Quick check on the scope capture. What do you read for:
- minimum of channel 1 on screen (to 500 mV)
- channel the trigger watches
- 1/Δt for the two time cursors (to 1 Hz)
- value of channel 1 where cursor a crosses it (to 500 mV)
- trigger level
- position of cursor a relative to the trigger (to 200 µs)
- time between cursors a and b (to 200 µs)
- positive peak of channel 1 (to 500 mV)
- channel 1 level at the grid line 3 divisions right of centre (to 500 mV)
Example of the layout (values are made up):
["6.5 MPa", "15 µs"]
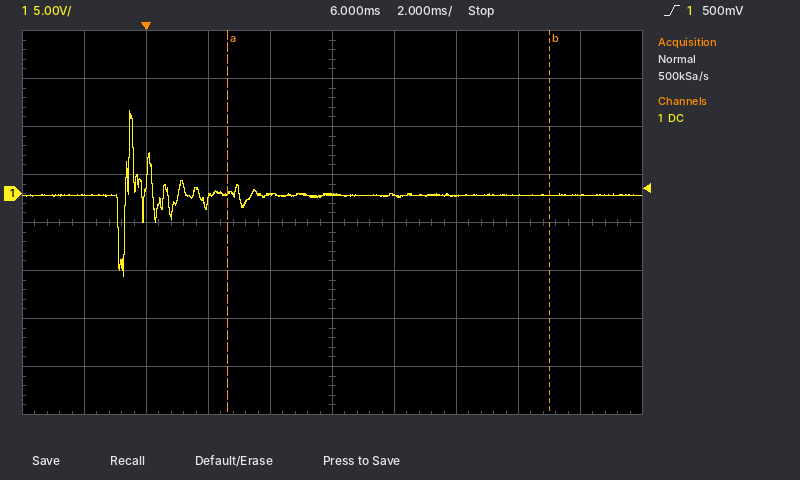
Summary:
["-8.5 V", "channel 1", "96 Hz", "0.0 V", "500 mV", "+2.6 ms", "10.4 ms", "8.5 V", "0.0 V"]
